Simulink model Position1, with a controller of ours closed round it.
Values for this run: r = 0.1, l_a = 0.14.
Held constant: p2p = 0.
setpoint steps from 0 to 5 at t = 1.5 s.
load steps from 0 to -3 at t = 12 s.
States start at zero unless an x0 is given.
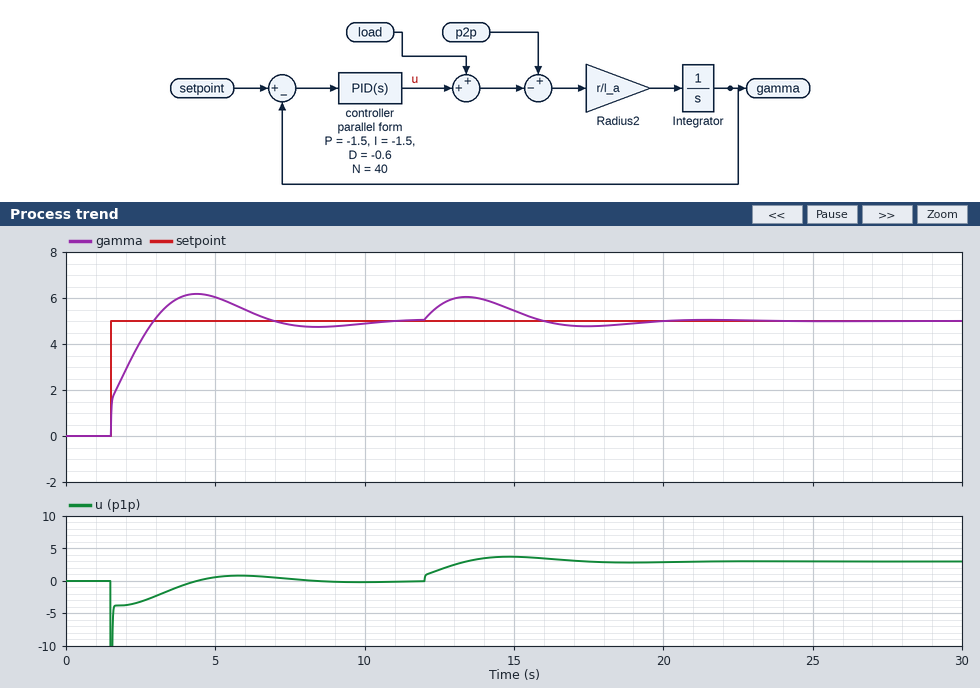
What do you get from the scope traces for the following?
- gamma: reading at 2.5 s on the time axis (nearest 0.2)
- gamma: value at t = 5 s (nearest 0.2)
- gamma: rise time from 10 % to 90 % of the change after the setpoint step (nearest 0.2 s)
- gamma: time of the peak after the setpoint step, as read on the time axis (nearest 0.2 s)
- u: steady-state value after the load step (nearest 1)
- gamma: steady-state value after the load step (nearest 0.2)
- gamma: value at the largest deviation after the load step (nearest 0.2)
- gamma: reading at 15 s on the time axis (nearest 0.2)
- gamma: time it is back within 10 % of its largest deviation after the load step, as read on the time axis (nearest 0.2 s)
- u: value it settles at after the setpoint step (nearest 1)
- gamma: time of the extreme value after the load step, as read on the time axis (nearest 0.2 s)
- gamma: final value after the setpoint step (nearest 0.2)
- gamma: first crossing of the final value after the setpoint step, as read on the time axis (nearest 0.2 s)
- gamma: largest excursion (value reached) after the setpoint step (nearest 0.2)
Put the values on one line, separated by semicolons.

4.2; 6.0; 1.2 s; 4.4 s; 3; 5.0; 6.0; 5.4; 19.0 s; 0; 13.4 s; 5.0; 3.0 s; 6.2
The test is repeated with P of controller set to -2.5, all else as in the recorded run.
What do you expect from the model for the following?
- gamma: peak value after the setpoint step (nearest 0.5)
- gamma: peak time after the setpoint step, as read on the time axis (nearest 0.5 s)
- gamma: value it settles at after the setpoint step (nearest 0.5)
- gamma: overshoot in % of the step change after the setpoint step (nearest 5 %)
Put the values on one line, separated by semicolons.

5.5; 4.0 s; 5.0; 15 %
